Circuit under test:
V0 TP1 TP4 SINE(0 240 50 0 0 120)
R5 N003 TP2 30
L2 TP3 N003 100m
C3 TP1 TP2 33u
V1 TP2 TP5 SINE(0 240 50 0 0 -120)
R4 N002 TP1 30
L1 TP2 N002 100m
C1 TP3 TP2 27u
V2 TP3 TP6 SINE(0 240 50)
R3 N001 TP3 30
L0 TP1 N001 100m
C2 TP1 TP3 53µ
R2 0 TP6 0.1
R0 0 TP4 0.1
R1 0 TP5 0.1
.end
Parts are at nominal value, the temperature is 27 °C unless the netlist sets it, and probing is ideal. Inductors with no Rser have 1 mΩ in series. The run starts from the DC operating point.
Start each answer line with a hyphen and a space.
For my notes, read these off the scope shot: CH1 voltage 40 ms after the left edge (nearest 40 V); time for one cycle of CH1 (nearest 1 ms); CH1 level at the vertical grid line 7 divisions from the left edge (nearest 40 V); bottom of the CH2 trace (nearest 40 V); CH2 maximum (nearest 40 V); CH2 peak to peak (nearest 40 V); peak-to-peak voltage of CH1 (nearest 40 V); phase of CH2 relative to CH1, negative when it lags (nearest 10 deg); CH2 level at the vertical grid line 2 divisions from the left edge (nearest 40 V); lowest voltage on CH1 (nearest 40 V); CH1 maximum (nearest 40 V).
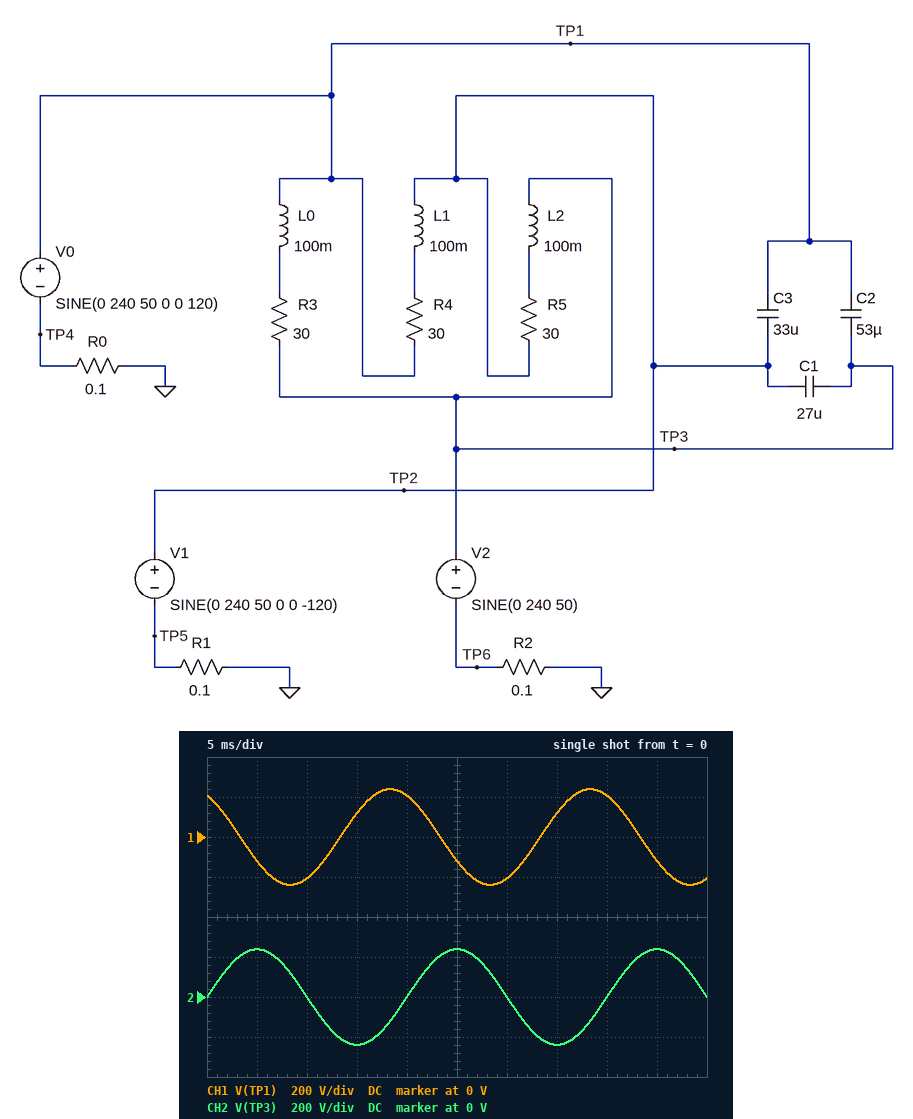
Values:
- 200 V
- 20 ms
- 120 V
- -240 V
- 240 V
- 480 V
- 480 V
- -120 deg
- 0 V
- -240 V
- 240 V
